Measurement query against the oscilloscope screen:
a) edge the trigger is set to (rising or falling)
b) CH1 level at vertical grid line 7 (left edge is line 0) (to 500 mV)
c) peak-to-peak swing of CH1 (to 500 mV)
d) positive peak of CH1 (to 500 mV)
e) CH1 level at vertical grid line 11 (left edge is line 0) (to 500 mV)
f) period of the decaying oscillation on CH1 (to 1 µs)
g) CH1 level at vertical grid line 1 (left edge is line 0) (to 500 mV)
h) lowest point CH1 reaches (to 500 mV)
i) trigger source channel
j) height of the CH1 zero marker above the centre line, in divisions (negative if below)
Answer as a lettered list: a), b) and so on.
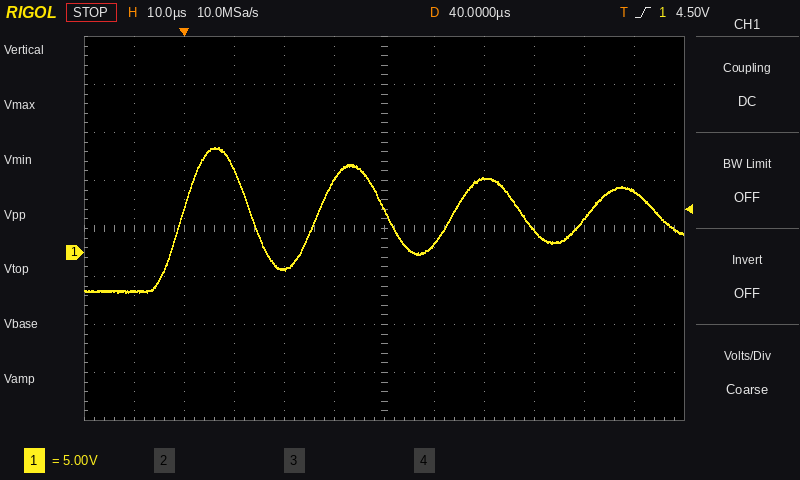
a) rising
b) 1.0 V
c) 15.0 V
d) 11.0 V
e) 6.5 V
f) 27 µs
g) -4.0 V
h) -4.0 V
i) CH1
j) -0.5 div
